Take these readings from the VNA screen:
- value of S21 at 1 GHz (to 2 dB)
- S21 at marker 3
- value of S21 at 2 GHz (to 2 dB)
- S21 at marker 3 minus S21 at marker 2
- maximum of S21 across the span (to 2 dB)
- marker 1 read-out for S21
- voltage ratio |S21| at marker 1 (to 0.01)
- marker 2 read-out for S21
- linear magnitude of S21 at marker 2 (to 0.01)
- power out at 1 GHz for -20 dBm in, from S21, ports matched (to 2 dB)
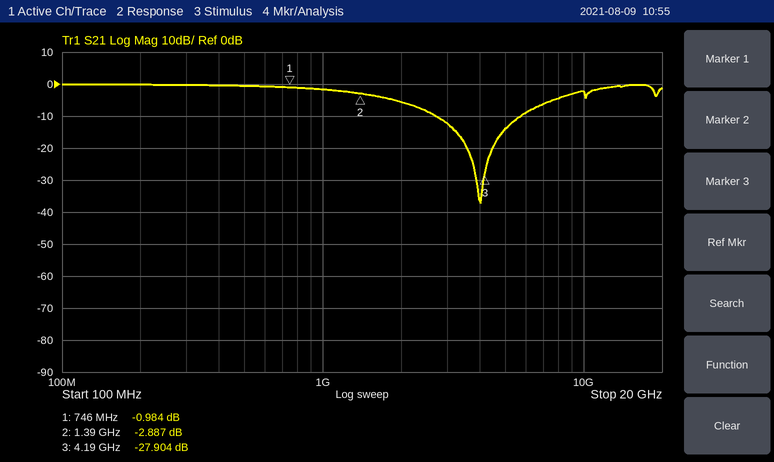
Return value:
-2 dB
-27.904 dB
-6 dB
-25.017 dB
0 dB
-0.984 dB
0.89
-2.887 dB
0.72
-22 dBm
